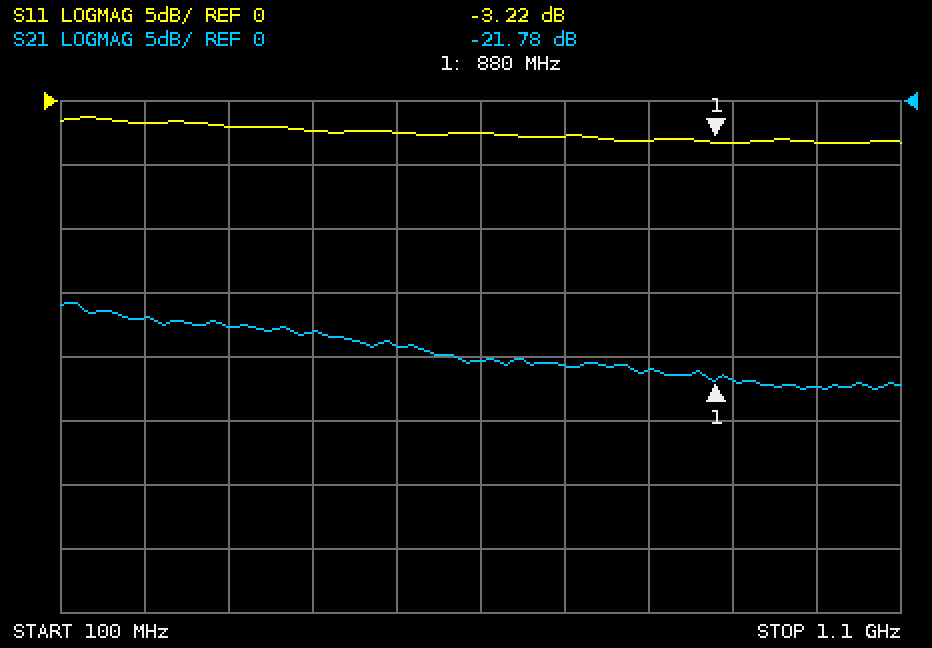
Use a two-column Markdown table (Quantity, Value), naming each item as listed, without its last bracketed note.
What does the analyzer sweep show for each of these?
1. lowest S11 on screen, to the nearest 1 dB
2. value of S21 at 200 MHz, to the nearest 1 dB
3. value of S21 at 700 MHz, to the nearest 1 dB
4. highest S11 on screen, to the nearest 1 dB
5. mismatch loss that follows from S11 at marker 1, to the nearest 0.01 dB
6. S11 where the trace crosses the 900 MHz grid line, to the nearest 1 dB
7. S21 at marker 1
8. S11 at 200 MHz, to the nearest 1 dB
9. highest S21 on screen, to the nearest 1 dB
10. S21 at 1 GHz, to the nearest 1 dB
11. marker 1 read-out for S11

| Quantity | Value |
|---|---|
| lowest S11 on screen, to the nearest 1 dB | -3 dB |
| value of S21 at 200 MHz, to the nearest 1 dB | -17 dB |
| value of S21 at 700 MHz, to the nearest 1 dB | -21 dB |
| highest S11 on screen, to the nearest 1 dB | -1 dB |
| mismatch loss that follows from S11 at marker 1, to the nearest 0.01 dB | 2.81 dB |
| S11 where the trace crosses the 900 MHz grid line, to the nearest 1 dB | -3 dB |
| S21 at marker 1 | -21.78 dB |
| S11 at 200 MHz, to the nearest 1 dB | -2 dB |
| highest S21 on screen, to the nearest 1 dB | -16 dB |
| S21 at 1 GHz, to the nearest 1 dB | -22 dB |
| marker 1 read-out for S11 | -3.22 dB |
